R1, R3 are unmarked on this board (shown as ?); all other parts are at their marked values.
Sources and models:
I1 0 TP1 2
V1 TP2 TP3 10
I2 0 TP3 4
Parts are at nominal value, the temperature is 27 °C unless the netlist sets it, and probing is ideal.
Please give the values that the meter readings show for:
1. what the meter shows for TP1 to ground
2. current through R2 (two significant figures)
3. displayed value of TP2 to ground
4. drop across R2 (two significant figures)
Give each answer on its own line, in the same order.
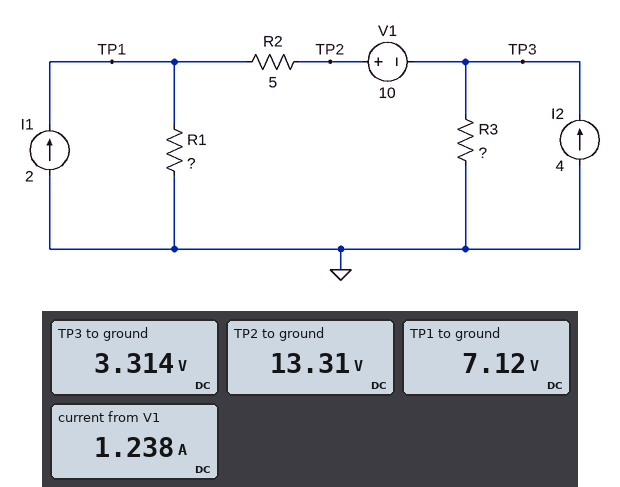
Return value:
7.12 V
1.2 A
13.31 V
6.2 V
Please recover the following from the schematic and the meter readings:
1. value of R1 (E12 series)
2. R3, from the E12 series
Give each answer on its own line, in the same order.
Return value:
2.2 Ω
1.2 Ω
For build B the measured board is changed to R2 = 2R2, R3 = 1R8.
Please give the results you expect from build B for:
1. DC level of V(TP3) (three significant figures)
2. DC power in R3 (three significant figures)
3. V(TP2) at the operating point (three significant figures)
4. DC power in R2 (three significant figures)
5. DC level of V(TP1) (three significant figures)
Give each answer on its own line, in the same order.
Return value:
3.48 V
6.74 W
13.5 V
9.38 W
8.94 V
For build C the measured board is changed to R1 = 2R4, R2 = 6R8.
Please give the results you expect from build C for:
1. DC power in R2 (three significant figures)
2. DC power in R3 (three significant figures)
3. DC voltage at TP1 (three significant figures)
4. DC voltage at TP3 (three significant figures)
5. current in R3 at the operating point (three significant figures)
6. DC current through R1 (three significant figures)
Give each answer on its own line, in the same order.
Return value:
6.29 W
11.1 W
7.11 V
3.65 V
3.04 A
2.96 A
